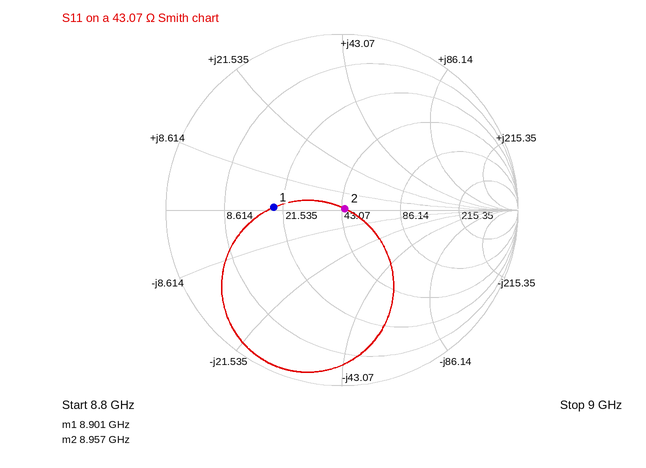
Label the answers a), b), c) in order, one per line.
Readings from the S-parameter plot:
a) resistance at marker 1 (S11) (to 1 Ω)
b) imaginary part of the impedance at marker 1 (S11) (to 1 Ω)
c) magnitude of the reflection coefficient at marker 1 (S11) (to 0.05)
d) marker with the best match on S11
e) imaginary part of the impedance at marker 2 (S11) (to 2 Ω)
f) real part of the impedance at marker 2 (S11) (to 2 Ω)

a) 19 Ω
b) +1 Ω
c) 0.40
d) marker 2
e) 0 Ω
f) 44 Ω
